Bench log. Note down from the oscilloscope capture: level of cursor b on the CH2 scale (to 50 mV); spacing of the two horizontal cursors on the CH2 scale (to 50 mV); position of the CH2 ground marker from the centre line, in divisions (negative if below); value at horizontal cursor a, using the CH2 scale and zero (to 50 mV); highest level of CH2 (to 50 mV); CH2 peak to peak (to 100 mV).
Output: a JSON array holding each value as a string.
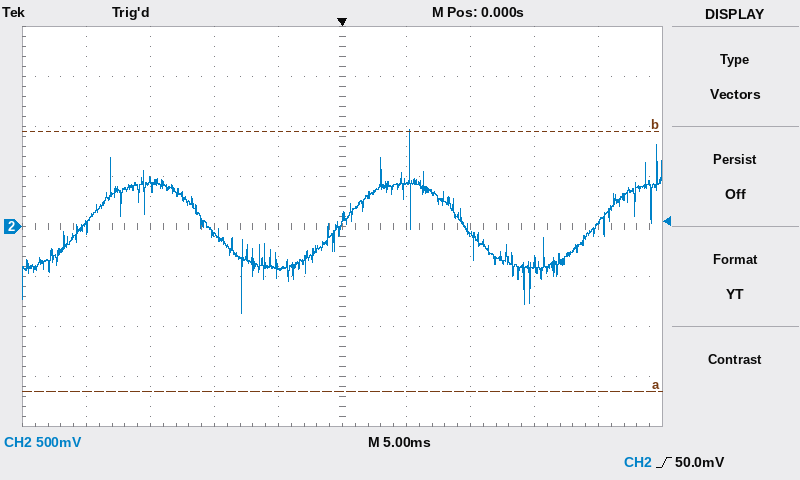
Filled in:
["950 mV", "2.60 V", "0.0 div", "-1.65 V", "950 mV", "1.80 V"]
